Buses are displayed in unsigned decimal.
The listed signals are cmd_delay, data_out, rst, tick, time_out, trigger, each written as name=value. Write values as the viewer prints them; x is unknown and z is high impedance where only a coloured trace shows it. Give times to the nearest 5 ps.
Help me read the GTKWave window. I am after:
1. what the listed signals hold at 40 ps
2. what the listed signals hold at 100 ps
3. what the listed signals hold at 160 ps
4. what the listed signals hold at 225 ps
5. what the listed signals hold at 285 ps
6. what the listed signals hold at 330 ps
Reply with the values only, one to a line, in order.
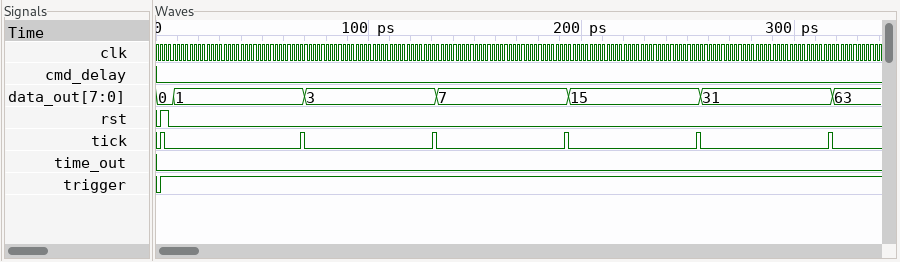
cmd_delay=0, data_out=1, rst=0, tick=0, time_out=0, trigger=1
cmd_delay=0, data_out=3, rst=0, tick=0, time_out=0, trigger=1
cmd_delay=0, data_out=7, rst=0, tick=0, time_out=0, trigger=1
cmd_delay=0, data_out=15, rst=0, tick=0, time_out=0, trigger=1
cmd_delay=0, data_out=31, rst=0, tick=0, time_out=0, trigger=1
cmd_delay=0, data_out=63, rst=0, tick=0, time_out=0, trigger=1
